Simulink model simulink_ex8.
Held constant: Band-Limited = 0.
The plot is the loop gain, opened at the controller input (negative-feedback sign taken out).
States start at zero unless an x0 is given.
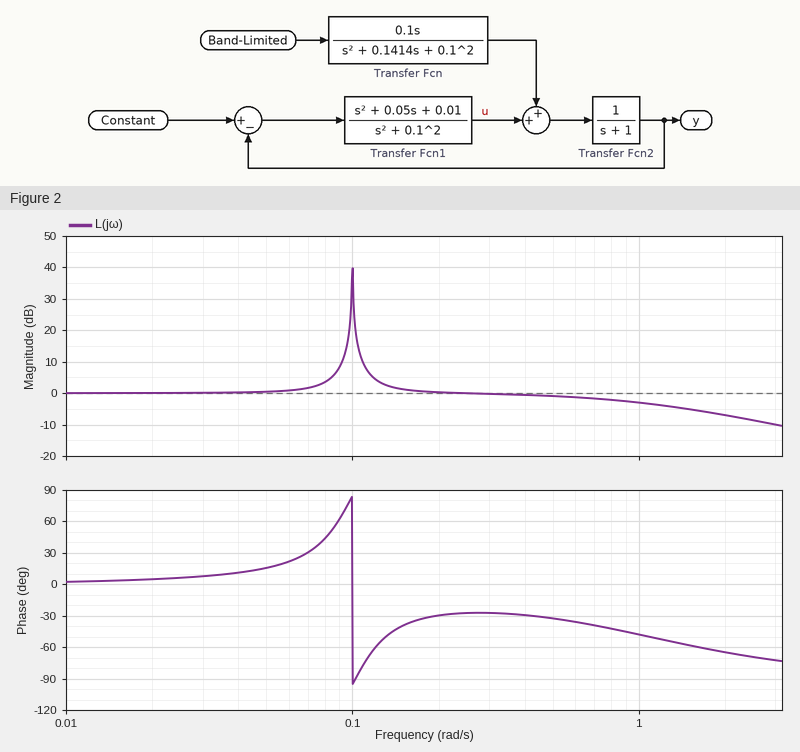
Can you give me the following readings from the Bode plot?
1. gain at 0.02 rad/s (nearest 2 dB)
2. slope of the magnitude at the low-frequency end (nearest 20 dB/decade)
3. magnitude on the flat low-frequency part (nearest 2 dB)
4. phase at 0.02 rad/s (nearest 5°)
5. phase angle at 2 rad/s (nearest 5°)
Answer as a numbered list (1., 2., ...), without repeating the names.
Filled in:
1. 0 dB
2. 0 dB/decade
3. 0 dB
4. 5°
5. -65°
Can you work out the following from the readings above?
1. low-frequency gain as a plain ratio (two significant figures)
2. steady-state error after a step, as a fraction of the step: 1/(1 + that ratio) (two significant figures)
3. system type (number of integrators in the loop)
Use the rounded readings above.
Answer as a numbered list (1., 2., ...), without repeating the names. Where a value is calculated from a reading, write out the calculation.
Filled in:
1. 10^(0 / 20) = 1.0
2. 1 / (1 + 1) = 0.50
3. 0
